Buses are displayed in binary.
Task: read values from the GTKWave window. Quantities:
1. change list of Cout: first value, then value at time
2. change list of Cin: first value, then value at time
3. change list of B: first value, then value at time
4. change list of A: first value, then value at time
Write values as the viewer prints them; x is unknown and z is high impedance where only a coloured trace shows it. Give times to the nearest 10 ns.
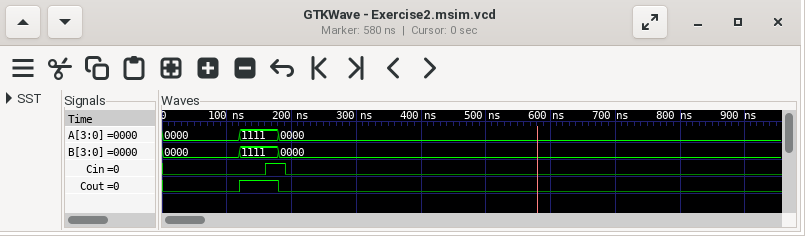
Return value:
0, 1 at 120 ns, 0 at 180 ns
0, 1 at 160 ns, 0 at 190 ns
0000, 1111 at 120 ns, 0000 at 180 ns
0000, 1111 at 120 ns, 0000 at 180 ns
